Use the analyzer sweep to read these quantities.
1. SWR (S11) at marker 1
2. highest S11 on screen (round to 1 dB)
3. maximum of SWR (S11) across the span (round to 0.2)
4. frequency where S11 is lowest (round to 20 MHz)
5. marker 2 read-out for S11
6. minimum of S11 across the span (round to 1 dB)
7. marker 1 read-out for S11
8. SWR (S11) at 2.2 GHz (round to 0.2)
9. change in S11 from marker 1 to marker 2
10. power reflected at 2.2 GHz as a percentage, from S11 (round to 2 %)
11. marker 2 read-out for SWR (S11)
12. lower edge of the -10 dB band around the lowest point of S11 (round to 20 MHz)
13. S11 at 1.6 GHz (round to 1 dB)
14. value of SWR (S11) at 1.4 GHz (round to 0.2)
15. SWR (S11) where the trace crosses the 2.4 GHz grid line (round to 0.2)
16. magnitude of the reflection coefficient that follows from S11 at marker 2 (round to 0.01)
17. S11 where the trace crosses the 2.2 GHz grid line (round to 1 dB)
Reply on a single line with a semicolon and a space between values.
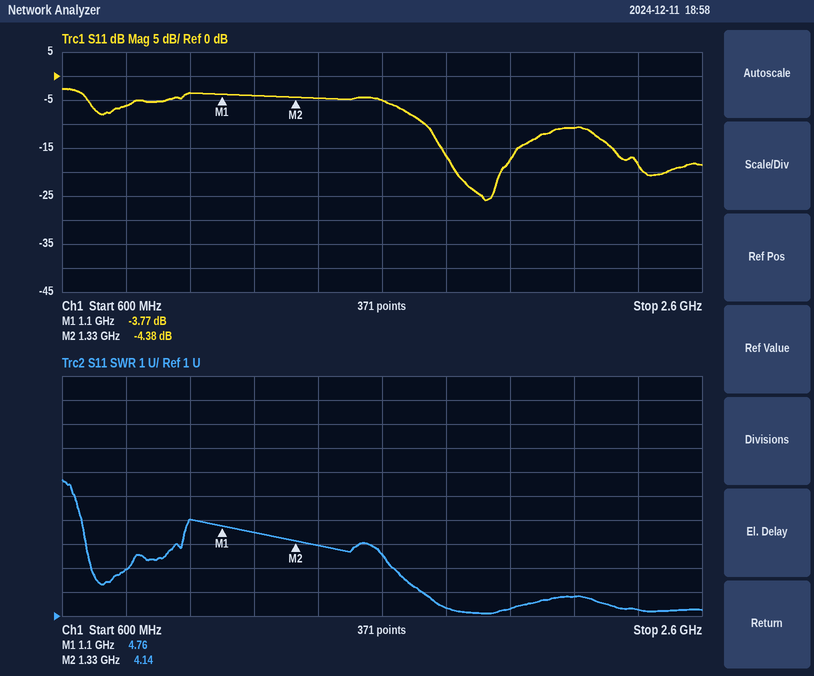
4.76; -3 dB; 6.6; 1.92 GHz; -4.38 dB; -26 dB; -3.77 dB; 1.8; -0.61 dB; 8 %; 4.14; 1.74 GHz; -5 dB; 4.0; 1.2; 0.60; -11 dB
